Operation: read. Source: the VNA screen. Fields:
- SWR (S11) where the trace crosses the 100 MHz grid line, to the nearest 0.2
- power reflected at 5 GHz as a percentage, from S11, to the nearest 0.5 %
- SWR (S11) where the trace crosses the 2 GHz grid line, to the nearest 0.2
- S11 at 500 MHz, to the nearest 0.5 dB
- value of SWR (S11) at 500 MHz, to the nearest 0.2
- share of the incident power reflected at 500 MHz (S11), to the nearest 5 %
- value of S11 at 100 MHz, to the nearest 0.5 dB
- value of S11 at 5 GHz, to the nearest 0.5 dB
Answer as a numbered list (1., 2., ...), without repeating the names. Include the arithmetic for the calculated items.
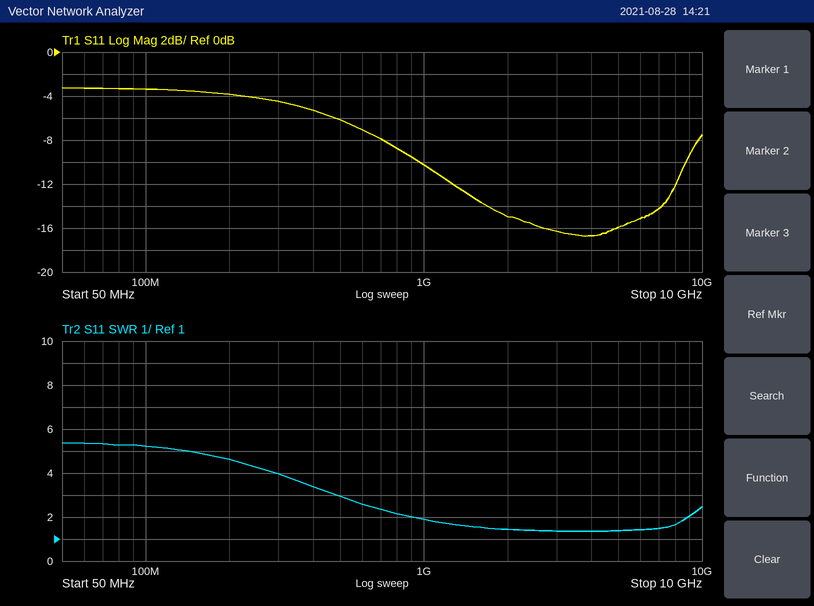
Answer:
1. 5.2
2. 10^(-16/10) ≈ 2.5 %
3. 1.4
4. -6.0 dB
5. 3.0
6. 10^(-6/10) ≈ 25 %
7. -3.5 dB
8. -16.0 dB
